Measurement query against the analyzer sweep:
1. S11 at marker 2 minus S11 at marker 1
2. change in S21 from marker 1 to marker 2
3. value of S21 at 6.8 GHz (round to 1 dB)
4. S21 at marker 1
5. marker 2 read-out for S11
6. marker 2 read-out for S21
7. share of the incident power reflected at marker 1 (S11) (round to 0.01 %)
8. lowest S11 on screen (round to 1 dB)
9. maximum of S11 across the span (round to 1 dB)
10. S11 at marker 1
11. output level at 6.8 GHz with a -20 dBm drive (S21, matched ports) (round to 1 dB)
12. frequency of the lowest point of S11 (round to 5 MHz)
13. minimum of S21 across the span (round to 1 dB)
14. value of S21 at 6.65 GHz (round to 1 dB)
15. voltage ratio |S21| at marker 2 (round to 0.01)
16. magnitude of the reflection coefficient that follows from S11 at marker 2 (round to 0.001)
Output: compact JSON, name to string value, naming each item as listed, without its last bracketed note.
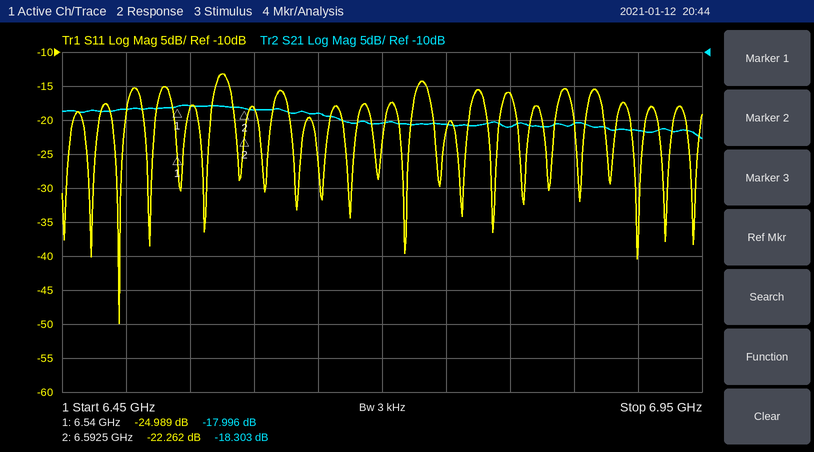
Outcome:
{"S11 at marker 2 minus S11 at marker 1": "2.727 dB", "change in S21 from marker 1 to marker 2": "-0.307 dB", "value of S21 at 6.8 GHz": "-21 dB", "S21 at marker 1": "-17.996 dB", "marker 2 read-out for S11": "-22.262 dB", "marker 2 read-out for S21": "-18.303 dB", "share of the incident power reflected at marker 1 (S11)": "0.32 %", "lowest S11 on screen": "-50 dB", "maximum of S11 across the span": "-13 dB", "S11 at marker 1": "-24.989 dB", "output level at 6.8 GHz with a -20 dBm drive (S21, matched ports)": "-41 dBm", "frequency of the lowest point of S11": "6.495 GHz", "minimum of S21 across the span": "-23 dB", "value of S21 at 6.65 GHz": "-19 dB", "voltage ratio |S21| at marker 2": "0.12", "magnitude of the reflection coefficient that follows from S11 at marker 2": "0.077"}
